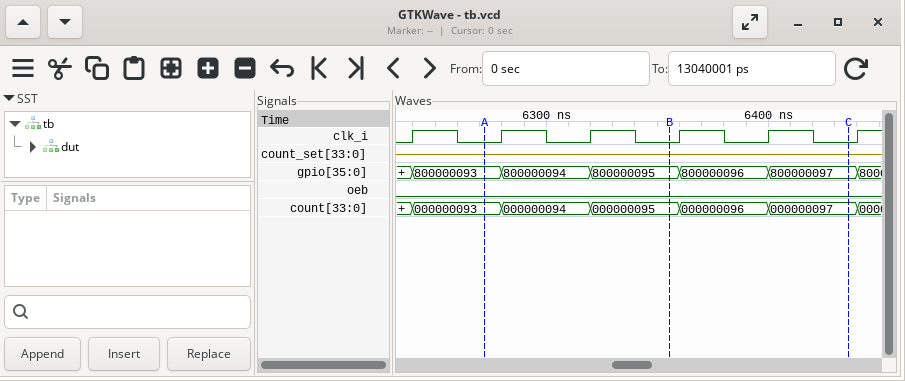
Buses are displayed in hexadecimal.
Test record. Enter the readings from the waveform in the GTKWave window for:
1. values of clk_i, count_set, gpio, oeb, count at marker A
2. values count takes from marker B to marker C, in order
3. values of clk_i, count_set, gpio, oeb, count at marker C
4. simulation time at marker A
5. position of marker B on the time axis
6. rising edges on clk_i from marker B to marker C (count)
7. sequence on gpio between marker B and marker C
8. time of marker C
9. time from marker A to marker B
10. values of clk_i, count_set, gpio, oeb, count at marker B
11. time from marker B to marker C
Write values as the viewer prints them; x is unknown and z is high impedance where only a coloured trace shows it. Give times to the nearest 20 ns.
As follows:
clk_i=0, count_set=z, gpio=800000093, oeb=0, count=000000093
000000095, 000000096, 000000097
clk_i=0, count_set=z, gpio=800000097, oeb=0, count=000000097
6280 ns
6360 ns
2
800000095, 800000096, 800000097
6440 ns
80 ns
clk_i=0, count_set=z, gpio=800000095, oeb=0, count=000000095
80 ns
